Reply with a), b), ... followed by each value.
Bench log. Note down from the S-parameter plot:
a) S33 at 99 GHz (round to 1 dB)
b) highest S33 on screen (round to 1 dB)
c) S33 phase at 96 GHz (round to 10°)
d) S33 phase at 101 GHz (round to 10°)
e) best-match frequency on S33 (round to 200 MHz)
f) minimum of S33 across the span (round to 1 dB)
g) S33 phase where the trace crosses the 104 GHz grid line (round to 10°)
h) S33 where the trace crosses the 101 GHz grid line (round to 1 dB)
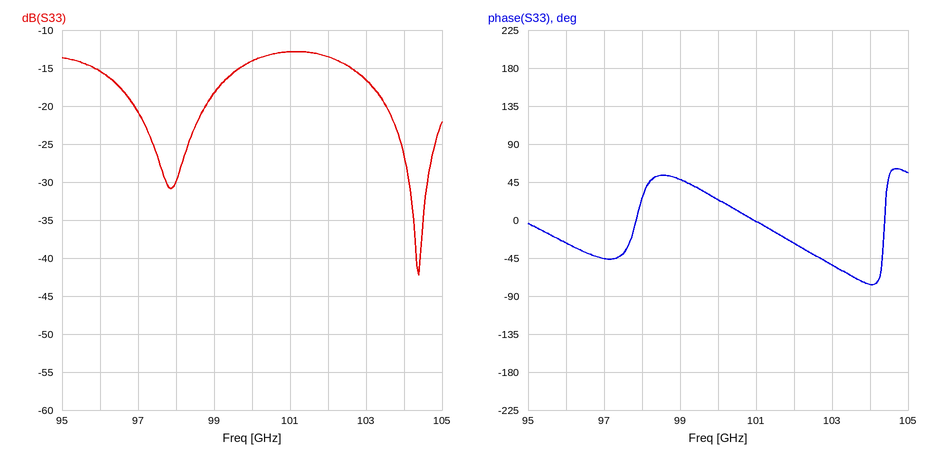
a) -18 dB
b) -13 dB
c) -30°
d) 0°
e) 104.4 GHz
f) -42 dB
g) -80°
h) -13 dB
